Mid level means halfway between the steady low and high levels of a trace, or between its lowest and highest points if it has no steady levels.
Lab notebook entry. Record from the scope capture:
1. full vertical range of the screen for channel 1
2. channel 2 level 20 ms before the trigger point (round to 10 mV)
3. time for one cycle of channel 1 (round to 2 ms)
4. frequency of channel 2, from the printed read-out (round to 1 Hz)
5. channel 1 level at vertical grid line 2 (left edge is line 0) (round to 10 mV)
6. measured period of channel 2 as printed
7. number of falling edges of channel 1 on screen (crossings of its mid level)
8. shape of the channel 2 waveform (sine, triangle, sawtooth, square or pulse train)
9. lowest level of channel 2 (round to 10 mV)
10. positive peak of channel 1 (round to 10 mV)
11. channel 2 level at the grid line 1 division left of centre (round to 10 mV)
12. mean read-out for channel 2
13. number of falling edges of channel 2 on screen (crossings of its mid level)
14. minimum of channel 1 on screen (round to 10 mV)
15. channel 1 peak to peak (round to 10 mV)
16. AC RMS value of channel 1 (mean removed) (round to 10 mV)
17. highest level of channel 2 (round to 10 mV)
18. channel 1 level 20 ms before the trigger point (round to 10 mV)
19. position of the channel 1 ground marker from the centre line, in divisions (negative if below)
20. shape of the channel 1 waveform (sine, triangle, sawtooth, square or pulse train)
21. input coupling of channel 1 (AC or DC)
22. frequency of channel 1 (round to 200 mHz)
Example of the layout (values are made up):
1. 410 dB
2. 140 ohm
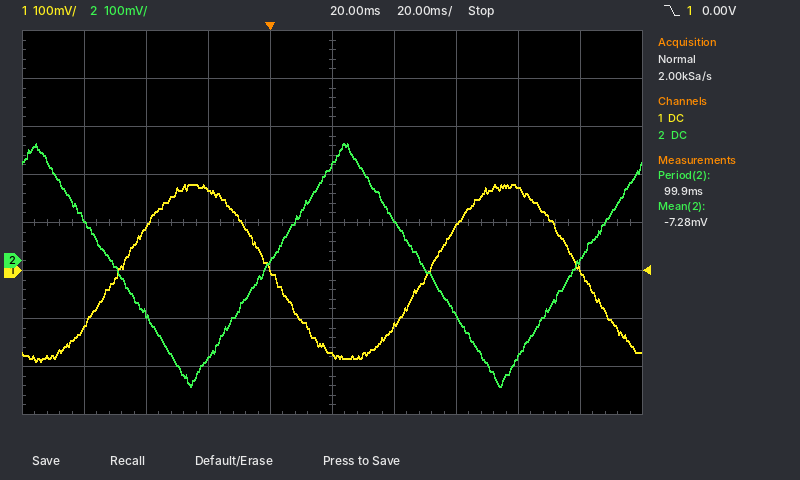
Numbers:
1. 800 mV
2. -200 mV
3. 100 ms
4. 10 Hz
5. 90 mV
6. 99.9 ms
7. 2
8. triangle
9. -260 mV
10. 180 mV
11. 0 mV
12. -7.28 mV
13. 2
14. -190 mV
15. 370 mV
16. 130 mV
17. 240 mV
18. 170 mV
19. -1.0 div
20. sine
21. DC
22. 10.0 Hz
